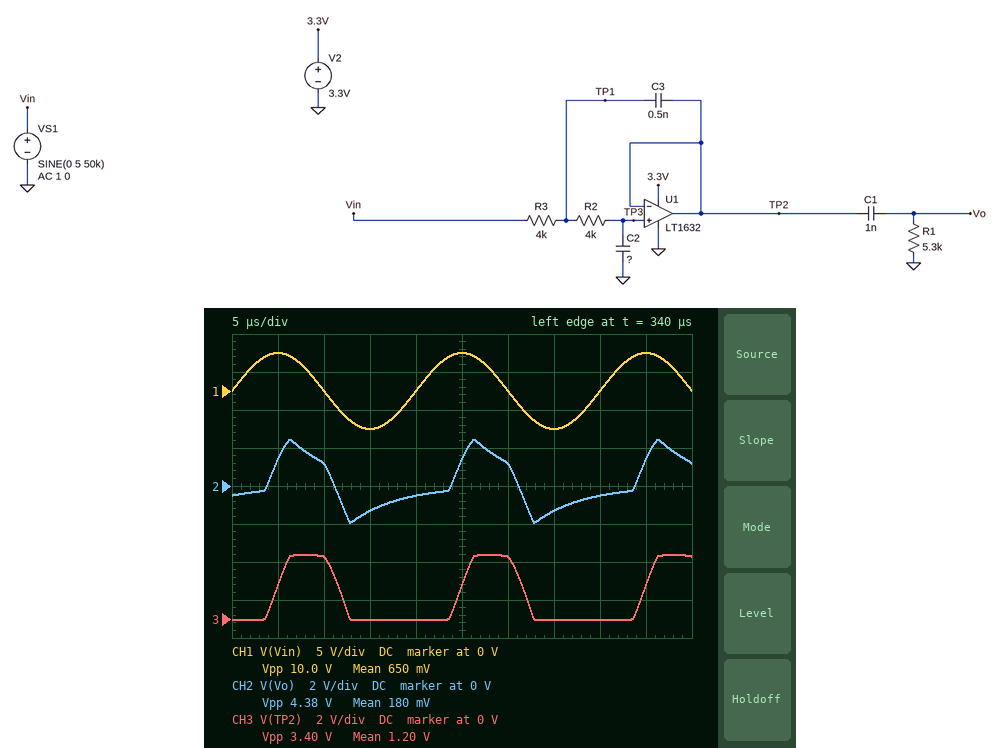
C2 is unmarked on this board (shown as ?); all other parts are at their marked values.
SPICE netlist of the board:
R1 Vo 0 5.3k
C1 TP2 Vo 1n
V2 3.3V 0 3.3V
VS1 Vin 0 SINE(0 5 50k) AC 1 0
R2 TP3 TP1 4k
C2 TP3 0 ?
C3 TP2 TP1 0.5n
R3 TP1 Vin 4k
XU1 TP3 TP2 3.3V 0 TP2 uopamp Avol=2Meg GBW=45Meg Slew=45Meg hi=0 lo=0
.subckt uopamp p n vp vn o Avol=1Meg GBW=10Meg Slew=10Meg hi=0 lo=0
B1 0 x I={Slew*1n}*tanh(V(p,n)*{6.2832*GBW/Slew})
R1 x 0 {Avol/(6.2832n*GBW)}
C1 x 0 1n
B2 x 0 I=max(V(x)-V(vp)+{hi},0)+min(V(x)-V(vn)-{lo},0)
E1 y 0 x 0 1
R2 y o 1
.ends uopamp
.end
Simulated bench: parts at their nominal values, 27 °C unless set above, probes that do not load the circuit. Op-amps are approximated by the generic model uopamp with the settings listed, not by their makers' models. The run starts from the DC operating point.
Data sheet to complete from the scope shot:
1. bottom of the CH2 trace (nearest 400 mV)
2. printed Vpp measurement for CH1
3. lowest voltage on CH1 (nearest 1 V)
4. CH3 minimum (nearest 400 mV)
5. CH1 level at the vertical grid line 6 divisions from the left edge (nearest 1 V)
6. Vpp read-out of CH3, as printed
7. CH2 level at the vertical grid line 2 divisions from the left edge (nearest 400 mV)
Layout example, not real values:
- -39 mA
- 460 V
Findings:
- -2.0 V
- 10.0 V
- -5 V
- 0 V
- 0 V
- 3.40 V
- 1.2 V
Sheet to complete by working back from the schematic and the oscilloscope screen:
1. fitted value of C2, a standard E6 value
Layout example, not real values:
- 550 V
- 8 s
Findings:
- 330 pF
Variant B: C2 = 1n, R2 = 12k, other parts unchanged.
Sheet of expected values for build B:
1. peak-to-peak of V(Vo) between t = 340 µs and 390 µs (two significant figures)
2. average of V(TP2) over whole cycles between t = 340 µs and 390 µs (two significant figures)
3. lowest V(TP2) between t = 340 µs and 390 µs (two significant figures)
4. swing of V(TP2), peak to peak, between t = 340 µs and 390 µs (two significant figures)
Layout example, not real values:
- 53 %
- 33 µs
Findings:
- 1.0 V
- 270 mV
- -45 mV
- 970 mV
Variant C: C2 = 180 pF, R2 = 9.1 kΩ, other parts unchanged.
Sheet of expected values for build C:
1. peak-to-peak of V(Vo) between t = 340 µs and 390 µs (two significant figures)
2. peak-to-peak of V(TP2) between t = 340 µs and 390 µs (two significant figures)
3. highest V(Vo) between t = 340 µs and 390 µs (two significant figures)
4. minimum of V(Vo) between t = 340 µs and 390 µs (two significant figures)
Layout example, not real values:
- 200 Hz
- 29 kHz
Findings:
- 4.5 V
- 3.4 V
- 2.5 V
- -2.0 V
